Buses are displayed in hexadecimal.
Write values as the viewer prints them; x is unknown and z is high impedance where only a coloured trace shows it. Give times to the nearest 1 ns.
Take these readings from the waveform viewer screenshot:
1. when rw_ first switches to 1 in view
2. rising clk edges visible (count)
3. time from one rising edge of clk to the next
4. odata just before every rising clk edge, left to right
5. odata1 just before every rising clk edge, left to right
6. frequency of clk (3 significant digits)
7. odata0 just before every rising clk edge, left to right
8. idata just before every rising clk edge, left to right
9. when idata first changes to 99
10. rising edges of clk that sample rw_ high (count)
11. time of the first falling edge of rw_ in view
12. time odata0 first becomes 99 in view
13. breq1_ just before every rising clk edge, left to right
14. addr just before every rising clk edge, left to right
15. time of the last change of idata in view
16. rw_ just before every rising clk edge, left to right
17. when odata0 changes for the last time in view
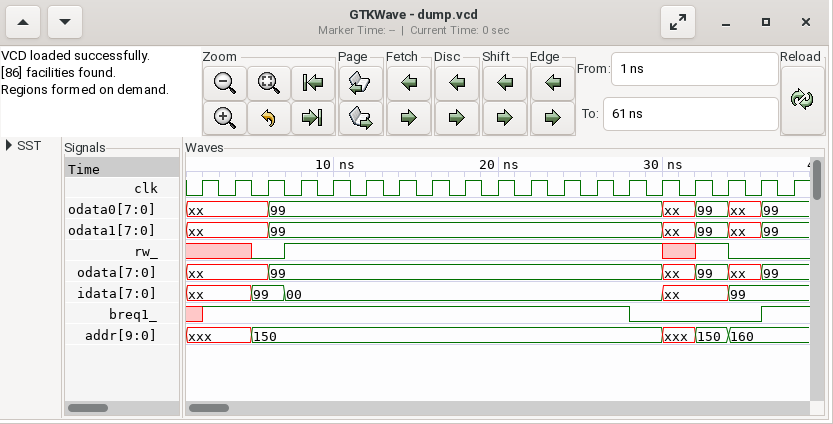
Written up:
7 ns
19
2 ns
xx, xx, xx, 99, 99, 99, 99, 99, 99, 99, 99, 99, 99, 99, 99, xx, 99, xx, 99
xx, xx, xx, 99, 99, 99, 99, 99, 99, 99, 99, 99, 99, 99, 99, xx, 99, xx, 99
500 MHz
xx, xx, xx, 99, 99, 99, 99, 99, 99, 99, 99, 99, 99, 99, 99, xx, 99, xx, 99
xx, xx, 99, 00, 00, 00, 00, 00, 00, 00, 00, 00, 00, 00, 00, xx, xx, 99, 99
5 ns
13
34 ns
6 ns
x 1 1 1 1 1 1 1 1 1 1 1 1 1 0 0 0 0 1
xxx, xxx, 150, 150, 150, 150, 150, 150, 150, 150, 150, 150, 150, 150, 150, xxx, 150, 160, 160
34 ns
x x 0 1 1 1 1 1 1 1 1 1 1 1 1 x 1 0 0
36 ns
